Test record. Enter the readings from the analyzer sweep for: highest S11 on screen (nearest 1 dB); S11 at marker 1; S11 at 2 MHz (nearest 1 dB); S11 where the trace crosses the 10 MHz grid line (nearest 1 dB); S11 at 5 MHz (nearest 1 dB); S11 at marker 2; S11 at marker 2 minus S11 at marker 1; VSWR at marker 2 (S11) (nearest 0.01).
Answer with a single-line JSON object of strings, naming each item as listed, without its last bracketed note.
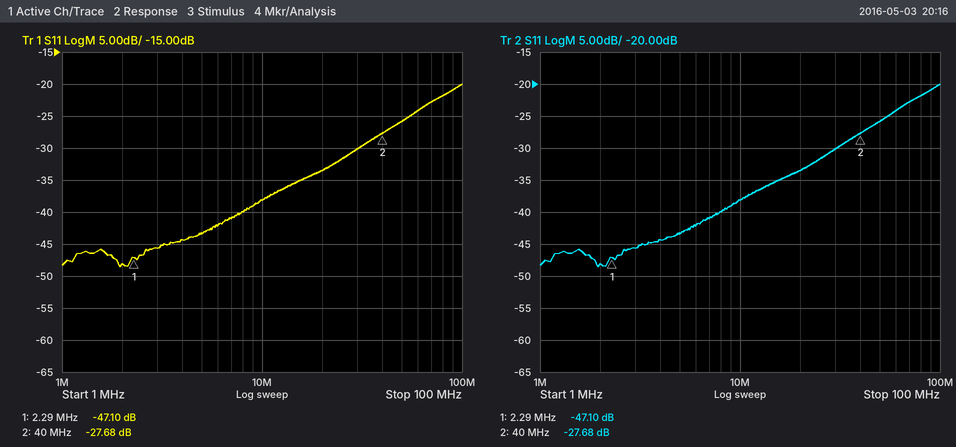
{"highest S11 on screen": "-20 dB", "S11 at marker 1": "-47.10 dB", "S11 at 2 MHz": "-48 dB", "S11 where the trace crosses the 10 MHz grid line": "-38 dB", "S11 at 5 MHz": "-43 dB", "S11 at marker 2": "-27.68 dB", "S11 at marker 2 minus S11 at marker 1": "19.42 dB", "VSWR at marker 2 (S11)": "1.09"}
